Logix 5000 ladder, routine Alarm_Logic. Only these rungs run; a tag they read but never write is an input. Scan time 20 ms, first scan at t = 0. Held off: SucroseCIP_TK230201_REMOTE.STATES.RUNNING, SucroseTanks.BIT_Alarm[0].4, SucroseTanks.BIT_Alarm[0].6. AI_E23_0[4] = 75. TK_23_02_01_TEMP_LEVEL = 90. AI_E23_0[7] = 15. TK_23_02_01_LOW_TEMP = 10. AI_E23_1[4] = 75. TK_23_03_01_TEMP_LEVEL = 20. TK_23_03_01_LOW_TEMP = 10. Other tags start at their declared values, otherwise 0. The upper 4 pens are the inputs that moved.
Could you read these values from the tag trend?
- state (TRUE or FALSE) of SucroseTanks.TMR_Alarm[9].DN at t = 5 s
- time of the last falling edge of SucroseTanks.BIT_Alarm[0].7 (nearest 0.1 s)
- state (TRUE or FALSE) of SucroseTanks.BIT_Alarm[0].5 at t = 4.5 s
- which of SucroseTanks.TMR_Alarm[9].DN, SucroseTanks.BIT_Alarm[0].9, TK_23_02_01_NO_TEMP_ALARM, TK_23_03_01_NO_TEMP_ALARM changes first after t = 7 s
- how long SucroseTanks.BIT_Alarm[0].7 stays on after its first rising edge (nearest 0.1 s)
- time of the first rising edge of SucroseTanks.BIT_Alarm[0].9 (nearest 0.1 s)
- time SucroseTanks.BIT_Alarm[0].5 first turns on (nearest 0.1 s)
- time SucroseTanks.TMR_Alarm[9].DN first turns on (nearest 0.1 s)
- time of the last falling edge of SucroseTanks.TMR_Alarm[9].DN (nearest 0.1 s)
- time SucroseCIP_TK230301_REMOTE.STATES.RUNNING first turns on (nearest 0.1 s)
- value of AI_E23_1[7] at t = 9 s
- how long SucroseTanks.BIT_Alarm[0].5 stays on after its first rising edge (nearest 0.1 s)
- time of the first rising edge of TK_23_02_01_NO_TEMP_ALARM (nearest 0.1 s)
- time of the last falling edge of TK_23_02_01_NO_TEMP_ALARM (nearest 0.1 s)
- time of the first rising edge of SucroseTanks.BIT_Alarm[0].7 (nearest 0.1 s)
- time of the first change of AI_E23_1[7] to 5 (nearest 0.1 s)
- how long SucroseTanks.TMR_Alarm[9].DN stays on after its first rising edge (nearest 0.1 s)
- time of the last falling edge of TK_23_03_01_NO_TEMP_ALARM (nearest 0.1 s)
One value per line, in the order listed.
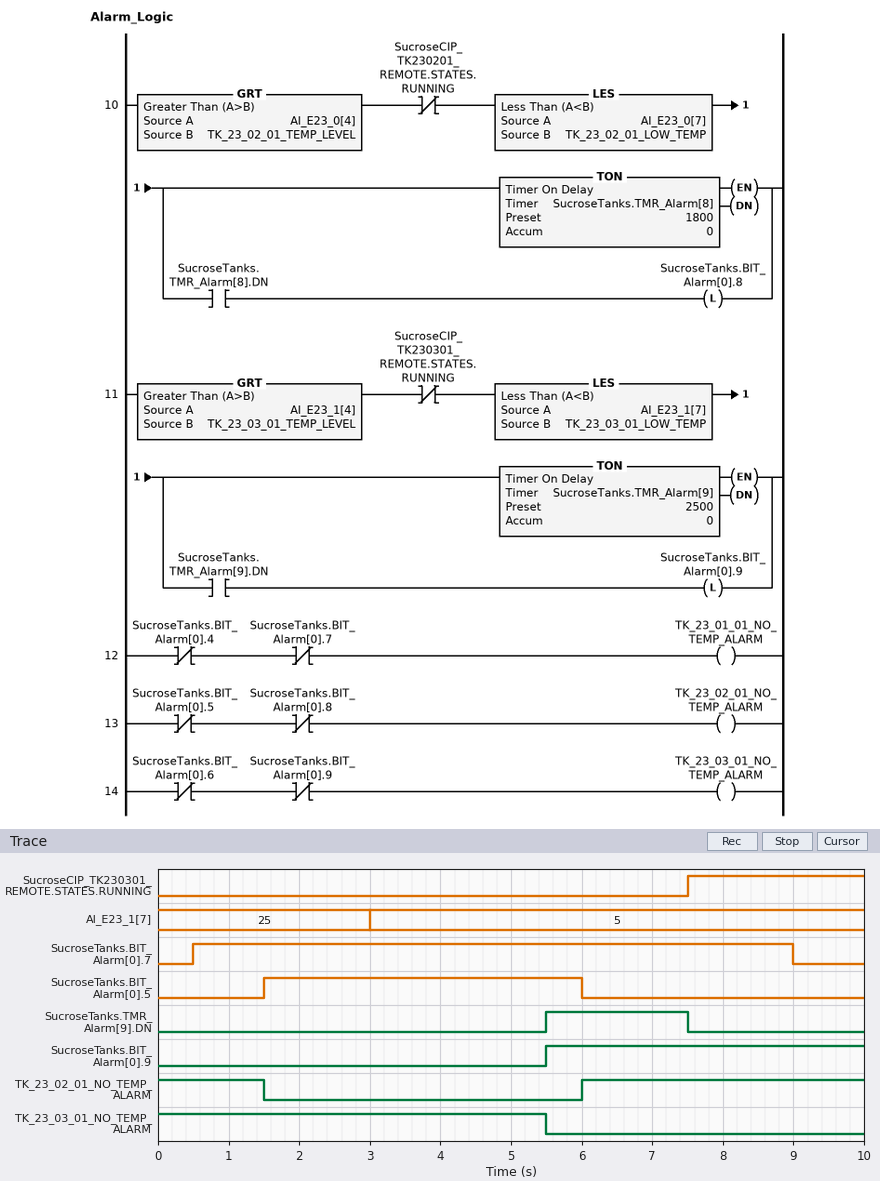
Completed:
FALSE
9.0 s
TRUE
SucroseTanks.TMR_Alarm[9].DN
8.5 s
5.5 s
1.5 s
5.5 s
7.5 s
7.5 s
5
4.5 s
6.0 s
1.5 s
0.5 s
3.0 s
2.0 s
5.5 s
